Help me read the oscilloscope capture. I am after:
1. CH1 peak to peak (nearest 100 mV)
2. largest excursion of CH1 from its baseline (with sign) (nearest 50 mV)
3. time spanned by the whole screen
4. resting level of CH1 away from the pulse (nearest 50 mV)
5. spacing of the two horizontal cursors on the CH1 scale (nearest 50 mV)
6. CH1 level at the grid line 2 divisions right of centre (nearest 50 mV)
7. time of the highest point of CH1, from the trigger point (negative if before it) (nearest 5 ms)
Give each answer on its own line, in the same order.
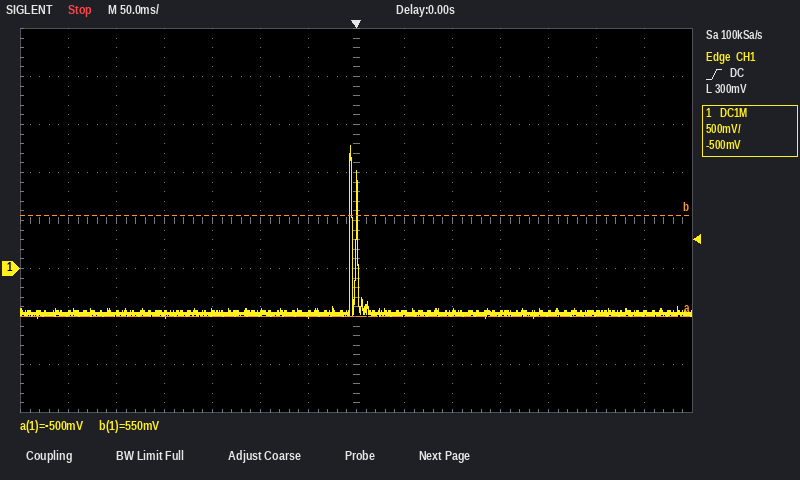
1.80 V
+1.75 V
700 ms
-450 mV
1.05 V
-450 mV
-5 ms
